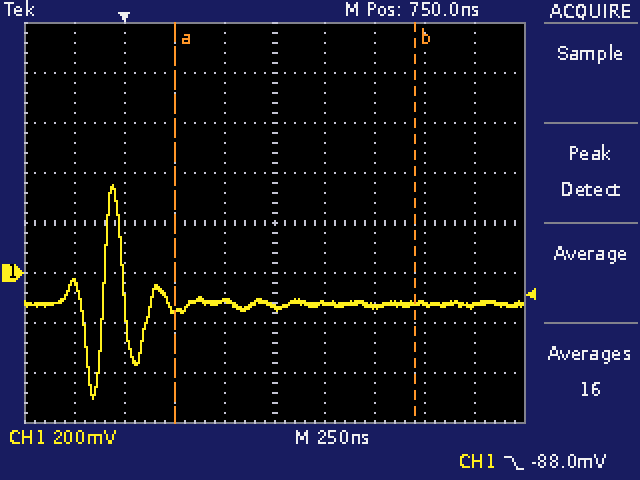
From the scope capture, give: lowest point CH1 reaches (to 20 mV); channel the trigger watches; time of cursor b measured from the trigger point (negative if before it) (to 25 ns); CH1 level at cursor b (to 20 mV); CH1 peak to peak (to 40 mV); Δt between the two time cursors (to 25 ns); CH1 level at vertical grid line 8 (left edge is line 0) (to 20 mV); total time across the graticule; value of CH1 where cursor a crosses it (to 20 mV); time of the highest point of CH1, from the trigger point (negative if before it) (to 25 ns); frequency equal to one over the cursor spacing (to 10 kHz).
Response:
-500 mV
CH1
+1.450 µs
-120 mV
840 mV
1.200 µs
-120 mV
2.5 µs
-140 mV
-50 ns
830 kHz
